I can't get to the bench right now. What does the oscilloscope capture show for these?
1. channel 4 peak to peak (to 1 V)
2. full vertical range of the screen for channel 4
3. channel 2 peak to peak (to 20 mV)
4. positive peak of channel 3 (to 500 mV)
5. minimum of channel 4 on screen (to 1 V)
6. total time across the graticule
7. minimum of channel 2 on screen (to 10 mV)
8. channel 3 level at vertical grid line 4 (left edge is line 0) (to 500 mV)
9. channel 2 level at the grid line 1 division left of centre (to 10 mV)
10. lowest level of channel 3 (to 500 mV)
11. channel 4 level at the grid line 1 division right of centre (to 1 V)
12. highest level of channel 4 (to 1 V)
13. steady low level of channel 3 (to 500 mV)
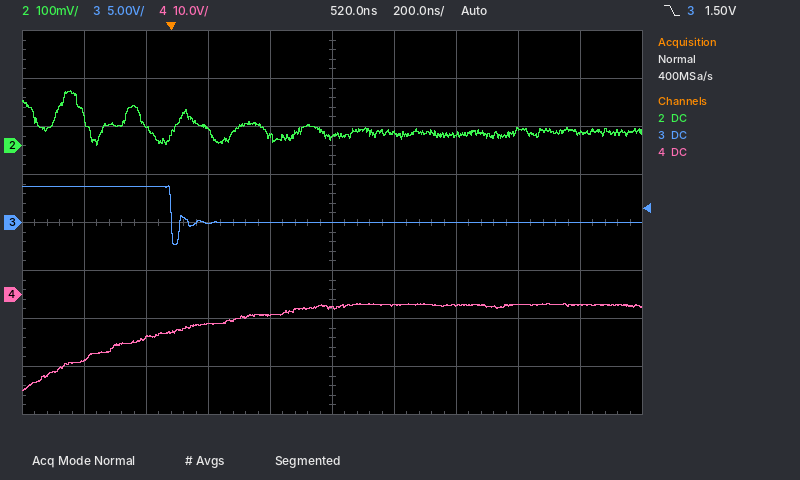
18 V
80 V
120 mV
4.0 V
-20 V
2 µs
0 mV
0.0 V
20 mV
-2.5 V
-2 V
-2 V
0.0 V
